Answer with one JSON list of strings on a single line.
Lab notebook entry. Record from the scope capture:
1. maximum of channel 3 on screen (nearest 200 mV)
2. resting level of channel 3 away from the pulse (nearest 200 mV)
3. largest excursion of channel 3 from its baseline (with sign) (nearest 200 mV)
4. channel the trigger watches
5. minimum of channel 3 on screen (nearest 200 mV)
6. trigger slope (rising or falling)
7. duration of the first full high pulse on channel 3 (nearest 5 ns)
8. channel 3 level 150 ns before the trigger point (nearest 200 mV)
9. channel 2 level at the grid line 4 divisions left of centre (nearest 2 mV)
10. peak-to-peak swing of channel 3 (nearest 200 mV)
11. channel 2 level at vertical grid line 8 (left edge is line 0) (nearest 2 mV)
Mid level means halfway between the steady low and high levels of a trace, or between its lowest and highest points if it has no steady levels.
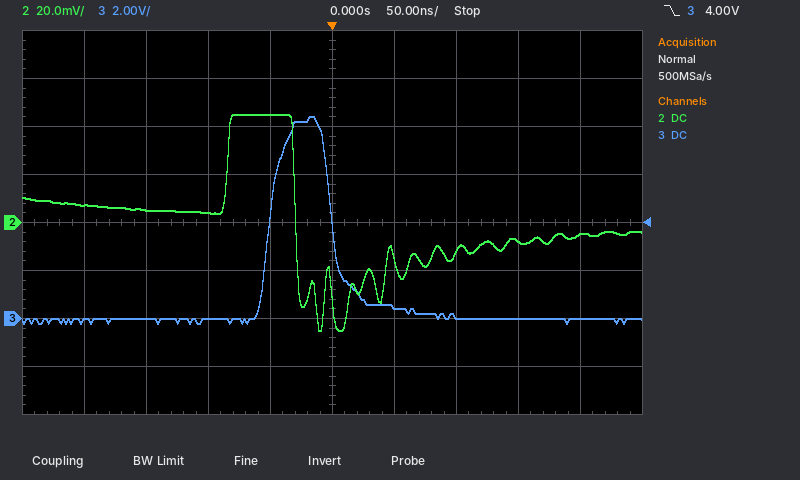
["8.4 V", "0.0 V", "+8.4 V", "channel 3", "-200 mV", "falling", "50 ns", "0.0 V", "8 mV", "8.6 V", "-8 mV"]
